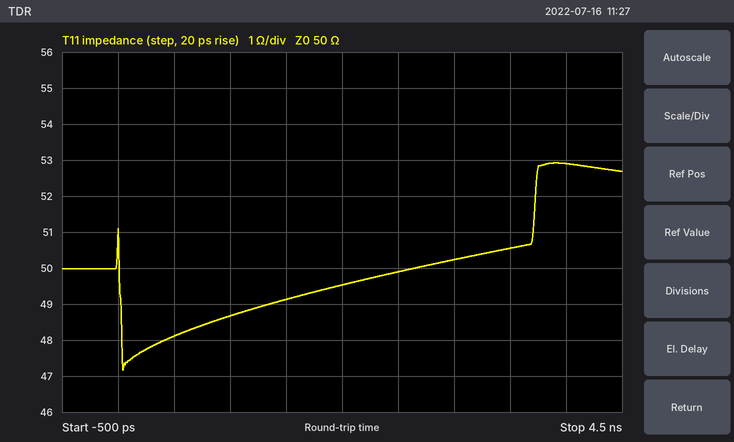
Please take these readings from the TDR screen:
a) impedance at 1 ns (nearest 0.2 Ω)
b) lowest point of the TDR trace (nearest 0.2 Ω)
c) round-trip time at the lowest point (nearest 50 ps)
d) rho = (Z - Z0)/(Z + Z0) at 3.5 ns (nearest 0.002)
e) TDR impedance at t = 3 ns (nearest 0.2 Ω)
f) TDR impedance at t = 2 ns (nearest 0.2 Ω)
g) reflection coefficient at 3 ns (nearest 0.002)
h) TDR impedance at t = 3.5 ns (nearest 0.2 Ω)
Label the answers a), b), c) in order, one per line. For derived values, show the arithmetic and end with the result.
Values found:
a) 48.6 Ω
b) 47.2 Ω
c) 50 ps
d) (50.6 − 50)/(50.6 + 50) ≈ +0.006
e) 50.2 Ω
f) 49.6 Ω
g) (50.2 − 50)/(50.2 + 50) ≈ +0.002
h) 50.6 Ω
